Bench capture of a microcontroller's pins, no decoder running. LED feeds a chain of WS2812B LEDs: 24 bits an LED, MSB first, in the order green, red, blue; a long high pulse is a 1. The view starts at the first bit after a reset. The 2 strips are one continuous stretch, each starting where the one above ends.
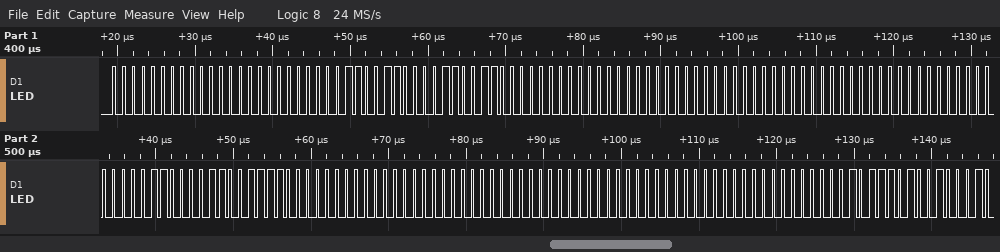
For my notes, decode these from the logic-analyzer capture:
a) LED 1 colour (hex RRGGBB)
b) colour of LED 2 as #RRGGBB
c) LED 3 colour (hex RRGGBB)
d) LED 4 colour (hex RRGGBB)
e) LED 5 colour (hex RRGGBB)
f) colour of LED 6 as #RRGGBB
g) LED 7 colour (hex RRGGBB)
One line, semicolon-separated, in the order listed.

#000000; #33CC00; #000000; #000000; #3CC300; #000000; #000000
